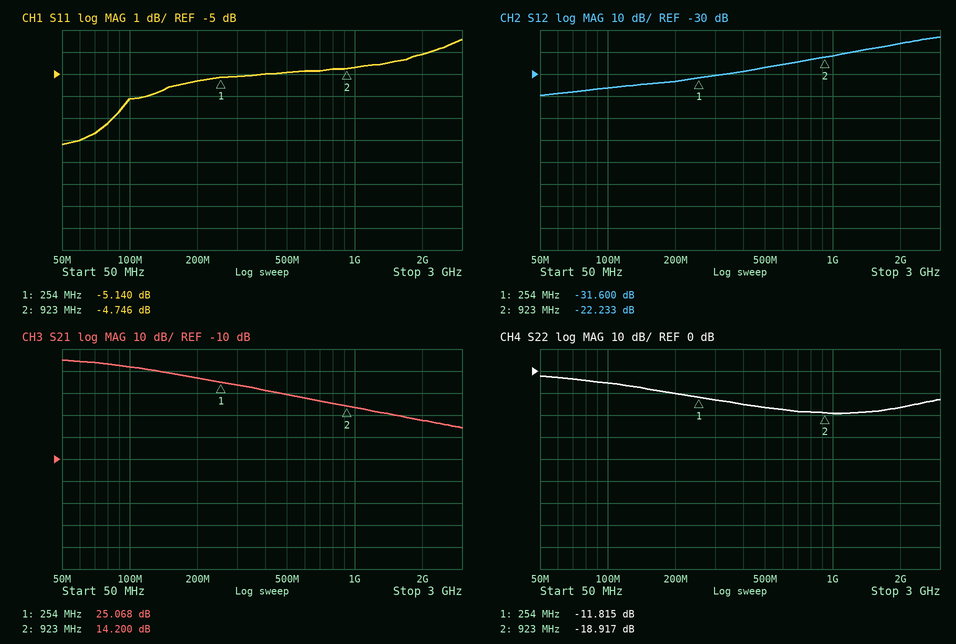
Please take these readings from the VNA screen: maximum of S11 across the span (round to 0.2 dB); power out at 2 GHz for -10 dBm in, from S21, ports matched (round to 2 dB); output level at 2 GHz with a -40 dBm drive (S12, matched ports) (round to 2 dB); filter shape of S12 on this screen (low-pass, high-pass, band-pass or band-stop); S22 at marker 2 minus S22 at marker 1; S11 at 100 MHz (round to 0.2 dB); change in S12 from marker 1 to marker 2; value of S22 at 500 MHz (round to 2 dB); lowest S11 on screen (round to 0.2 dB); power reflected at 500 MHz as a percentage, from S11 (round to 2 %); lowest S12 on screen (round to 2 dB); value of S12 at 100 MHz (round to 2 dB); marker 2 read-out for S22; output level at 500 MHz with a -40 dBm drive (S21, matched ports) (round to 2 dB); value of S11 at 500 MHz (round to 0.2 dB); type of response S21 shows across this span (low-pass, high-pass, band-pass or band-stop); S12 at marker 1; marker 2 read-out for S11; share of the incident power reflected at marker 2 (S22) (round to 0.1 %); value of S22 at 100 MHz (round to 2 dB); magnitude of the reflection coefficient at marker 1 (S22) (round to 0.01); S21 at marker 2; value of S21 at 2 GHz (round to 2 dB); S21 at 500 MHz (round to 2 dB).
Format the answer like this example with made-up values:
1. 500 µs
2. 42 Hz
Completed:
1. -3.4 dB
2. -2 dBm
3. -56 dBm
4. high-pass
5. -7.102 dB
6. -6.2 dB
7. 9.367 dB
8. -16 dB
9. -8.2 dB
10. 32 %
11. -40 dB
12. -36 dB
13. -18.917 dB
14. -20 dBm
15. -5.0 dB
16. low-pass
17. -31.600 dB
18. -4.746 dB
19. 1.3 %
20. -6 dB
21. 0.26
22. 14.200 dB
23. 8 dB
24. 20 dB
